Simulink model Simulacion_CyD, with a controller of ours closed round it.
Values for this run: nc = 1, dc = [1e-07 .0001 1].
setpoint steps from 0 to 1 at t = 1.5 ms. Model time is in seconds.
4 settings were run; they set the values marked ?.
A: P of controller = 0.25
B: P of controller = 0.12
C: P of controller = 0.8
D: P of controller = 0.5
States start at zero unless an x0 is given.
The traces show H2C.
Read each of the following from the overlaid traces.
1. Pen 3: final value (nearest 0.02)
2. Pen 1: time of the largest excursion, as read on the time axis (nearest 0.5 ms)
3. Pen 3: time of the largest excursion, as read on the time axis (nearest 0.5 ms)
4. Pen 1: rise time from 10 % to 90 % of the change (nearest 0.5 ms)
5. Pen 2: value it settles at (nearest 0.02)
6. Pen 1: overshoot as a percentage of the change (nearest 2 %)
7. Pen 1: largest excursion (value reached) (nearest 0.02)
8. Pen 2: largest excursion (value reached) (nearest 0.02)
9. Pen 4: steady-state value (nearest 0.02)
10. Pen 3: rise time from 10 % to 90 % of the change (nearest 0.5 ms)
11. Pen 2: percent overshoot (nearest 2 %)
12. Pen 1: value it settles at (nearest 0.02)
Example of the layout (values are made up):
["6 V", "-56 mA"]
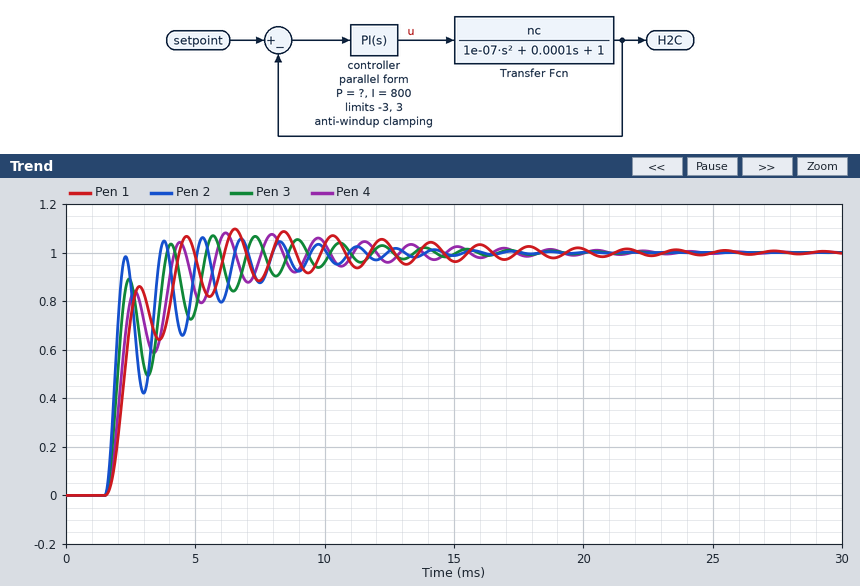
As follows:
["1.00", "6.5 ms", "5.5 ms", "2.5 ms", "1.00", "10 %", "1.10", "1.06", "1.00", "2.0 ms", "6 %", "1.00"]
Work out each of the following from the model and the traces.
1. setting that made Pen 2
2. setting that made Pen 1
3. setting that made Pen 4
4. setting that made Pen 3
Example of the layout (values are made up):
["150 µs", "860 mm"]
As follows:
["C", "B", "A", "D"]
